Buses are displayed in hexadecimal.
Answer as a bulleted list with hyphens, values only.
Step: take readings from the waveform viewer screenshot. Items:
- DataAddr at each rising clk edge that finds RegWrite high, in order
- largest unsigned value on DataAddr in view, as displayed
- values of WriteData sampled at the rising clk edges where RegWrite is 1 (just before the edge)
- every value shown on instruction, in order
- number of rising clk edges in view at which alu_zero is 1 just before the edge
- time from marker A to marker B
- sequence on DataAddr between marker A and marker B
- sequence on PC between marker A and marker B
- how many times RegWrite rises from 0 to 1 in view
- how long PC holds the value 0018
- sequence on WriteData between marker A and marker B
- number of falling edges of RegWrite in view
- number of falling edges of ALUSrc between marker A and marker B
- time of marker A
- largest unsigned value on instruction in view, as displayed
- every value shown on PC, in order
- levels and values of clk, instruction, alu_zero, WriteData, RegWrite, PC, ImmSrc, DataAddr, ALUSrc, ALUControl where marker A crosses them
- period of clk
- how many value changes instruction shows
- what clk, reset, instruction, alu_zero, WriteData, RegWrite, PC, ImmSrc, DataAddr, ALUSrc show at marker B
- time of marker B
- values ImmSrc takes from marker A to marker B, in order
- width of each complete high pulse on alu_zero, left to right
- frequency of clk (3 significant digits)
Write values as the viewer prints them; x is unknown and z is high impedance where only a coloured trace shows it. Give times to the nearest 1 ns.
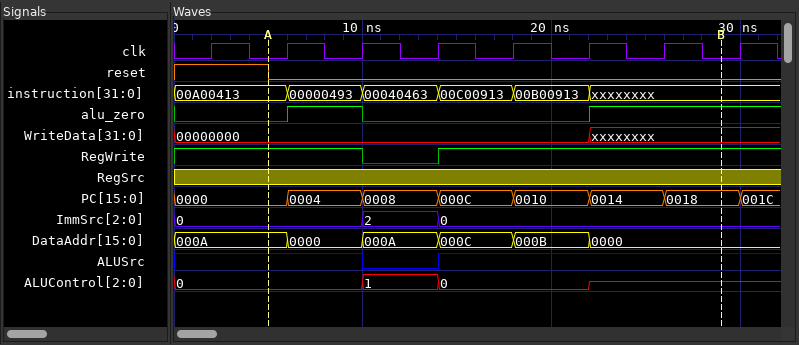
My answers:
- 000A, 000A, 0000, 000C, 000B, 0000, 0000
- 000C
- 00000000, 00000000, 00000000, 00000000, 00000000, xxxxxxxx, xxxxxxxx
- 00A00413, 00000493, 00040463, 00C00913, 00B00913, xxxxxxxx
- 3
- 24 ns
- 000A, 0000, 000A, 000C, 000B, 0000
- 0000, 0004, 0008, 000C, 0010, 0014, 0018
- 1
- 4 ns
- 00000000, xxxxxxxx
- 1
- 1
- 5 ns
- 00C00913
- 0000, 0004, 0008, 000C, 0010, 0014, 0018, 001C
- clk=0, instruction=00A00413, alu_zero=0, WriteData=00000000, RegWrite=1, PC=0000, ImmSrc=0, DataAddr=000A, ALUSrc=1, ALUControl=0
- 4 ns
- 5
- clk=0, reset=0, instruction=xxxxxxxx, alu_zero=1, WriteData=xxxxxxxx, RegWrite=1, PC=0018, ImmSrc=0, DataAddr=0000, ALUSrc=1
- 29 ns
- 0, 2, 0
- 4 ns
- 250 MHz
